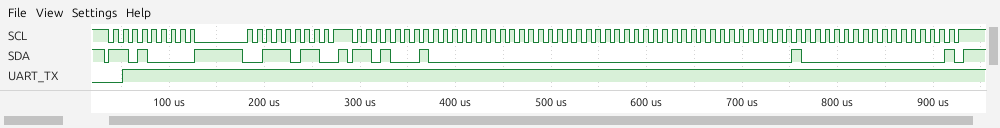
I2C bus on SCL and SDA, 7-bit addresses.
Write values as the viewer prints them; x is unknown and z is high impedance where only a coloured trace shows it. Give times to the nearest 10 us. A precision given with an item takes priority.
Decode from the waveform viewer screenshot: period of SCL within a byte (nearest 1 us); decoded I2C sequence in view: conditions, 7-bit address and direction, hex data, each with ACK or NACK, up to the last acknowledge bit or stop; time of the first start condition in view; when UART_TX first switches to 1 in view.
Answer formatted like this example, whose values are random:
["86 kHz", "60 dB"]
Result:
["10 us", "start, address 68 write ACK, 3B ACK, stop, start, address 68 read ACK, 00 ACK, 00 ACK, 00 ACK, 00 ACK, 40 ACK, 00 NACK, stop", "30 us", "50 us"]
